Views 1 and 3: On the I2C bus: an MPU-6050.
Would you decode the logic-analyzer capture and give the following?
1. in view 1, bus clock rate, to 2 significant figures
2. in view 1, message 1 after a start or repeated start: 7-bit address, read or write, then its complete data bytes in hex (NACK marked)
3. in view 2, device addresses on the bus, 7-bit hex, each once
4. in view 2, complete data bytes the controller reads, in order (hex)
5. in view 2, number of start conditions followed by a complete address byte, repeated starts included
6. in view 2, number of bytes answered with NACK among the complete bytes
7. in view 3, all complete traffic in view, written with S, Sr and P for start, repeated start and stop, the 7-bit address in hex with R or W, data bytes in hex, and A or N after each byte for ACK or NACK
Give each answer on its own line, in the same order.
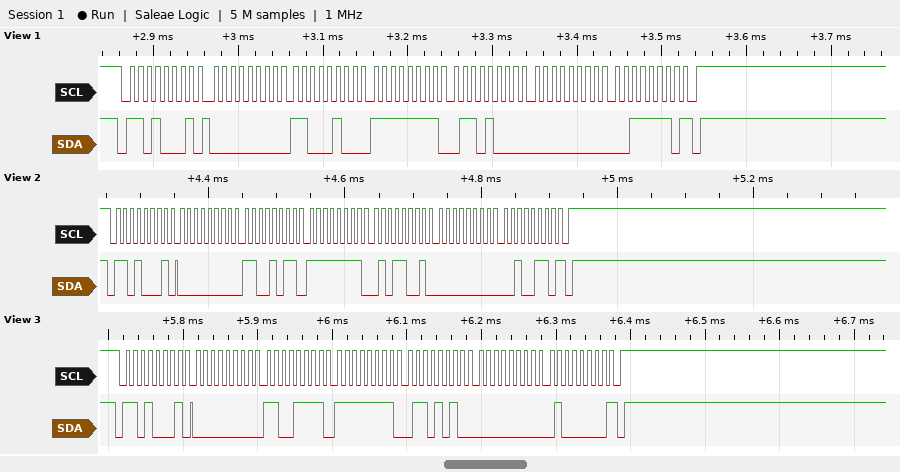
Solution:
100 kHz
0x68 read: 00 C4 FF 68 00 3E NACK
0x68
00 CB FF 59 00 26
1
1
S 68R A 00 A CF A FF A 6A A 00 A 40 N P
